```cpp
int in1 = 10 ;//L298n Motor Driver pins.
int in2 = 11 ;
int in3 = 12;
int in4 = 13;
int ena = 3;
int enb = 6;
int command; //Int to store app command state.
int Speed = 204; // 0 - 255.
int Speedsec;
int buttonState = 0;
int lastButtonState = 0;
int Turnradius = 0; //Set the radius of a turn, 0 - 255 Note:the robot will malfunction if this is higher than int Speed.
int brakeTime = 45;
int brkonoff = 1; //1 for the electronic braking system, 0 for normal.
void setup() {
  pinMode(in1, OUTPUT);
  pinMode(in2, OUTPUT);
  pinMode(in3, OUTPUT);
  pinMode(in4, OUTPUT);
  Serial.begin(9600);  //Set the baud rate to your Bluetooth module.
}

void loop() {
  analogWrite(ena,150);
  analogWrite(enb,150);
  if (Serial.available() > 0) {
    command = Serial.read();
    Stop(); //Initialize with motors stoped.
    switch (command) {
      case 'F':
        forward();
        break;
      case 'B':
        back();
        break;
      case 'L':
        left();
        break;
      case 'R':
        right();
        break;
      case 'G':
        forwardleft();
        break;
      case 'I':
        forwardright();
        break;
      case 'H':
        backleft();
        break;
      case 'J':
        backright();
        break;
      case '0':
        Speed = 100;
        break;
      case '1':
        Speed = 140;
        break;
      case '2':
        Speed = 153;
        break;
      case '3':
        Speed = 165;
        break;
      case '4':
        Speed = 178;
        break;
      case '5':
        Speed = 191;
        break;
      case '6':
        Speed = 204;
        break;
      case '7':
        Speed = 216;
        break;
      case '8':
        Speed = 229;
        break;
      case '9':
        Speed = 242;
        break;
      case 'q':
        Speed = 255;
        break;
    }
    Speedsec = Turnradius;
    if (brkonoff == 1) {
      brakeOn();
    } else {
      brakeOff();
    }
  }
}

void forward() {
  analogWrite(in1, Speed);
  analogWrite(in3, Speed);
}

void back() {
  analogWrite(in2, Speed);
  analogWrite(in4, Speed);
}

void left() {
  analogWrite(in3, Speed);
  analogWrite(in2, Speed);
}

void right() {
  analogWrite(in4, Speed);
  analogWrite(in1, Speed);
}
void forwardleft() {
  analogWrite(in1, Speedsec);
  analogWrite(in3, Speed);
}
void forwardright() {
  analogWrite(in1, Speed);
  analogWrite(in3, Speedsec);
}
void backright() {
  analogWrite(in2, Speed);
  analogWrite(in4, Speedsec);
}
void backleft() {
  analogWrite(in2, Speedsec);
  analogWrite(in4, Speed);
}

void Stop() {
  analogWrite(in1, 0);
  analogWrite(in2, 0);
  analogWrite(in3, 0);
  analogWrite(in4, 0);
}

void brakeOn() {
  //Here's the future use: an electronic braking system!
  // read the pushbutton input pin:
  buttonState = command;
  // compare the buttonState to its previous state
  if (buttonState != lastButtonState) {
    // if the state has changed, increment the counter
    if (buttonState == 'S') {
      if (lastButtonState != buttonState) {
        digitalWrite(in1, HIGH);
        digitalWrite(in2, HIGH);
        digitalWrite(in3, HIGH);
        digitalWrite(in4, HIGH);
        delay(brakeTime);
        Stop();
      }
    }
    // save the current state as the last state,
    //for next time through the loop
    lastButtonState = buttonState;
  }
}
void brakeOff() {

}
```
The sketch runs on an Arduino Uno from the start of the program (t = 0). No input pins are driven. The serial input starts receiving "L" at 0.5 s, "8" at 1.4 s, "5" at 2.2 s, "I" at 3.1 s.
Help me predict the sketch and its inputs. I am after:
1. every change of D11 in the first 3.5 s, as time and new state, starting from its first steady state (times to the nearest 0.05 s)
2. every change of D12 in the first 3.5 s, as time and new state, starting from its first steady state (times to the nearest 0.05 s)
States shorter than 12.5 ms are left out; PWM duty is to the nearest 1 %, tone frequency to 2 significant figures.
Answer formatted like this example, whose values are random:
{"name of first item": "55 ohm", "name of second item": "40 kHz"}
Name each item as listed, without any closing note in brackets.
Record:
{"every change of D11 in the first 3.5 s, as time and new state, starting from its first steady state": "0 s low; 0.5 s PWM 80 %; 1.4 s low", "every change of D12 in the first 3.5 s, as time and new state, starting from its first steady state": "0 s low; 0.5 s high; 1.4 s low"}
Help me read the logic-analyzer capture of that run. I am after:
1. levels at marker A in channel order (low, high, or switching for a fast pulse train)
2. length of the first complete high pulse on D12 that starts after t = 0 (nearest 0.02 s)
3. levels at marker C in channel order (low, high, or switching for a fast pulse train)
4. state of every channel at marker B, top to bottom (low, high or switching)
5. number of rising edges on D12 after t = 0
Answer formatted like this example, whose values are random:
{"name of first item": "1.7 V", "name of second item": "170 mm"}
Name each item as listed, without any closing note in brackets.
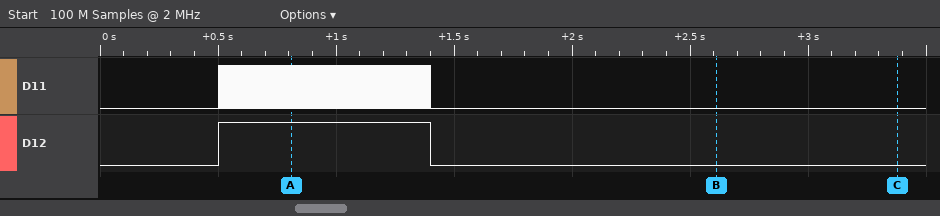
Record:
{"levels at marker A in channel order": "D11 switching, D12 high", "length of the first complete high pulse on D12 that starts after t = 0": "0.90 s", "levels at marker C in channel order": "D11 low, D12 low", "state of every channel at marker B, top to bottom": "D11 low, D12 low", "number of rising edges on D12 after t = 0": "1"}
